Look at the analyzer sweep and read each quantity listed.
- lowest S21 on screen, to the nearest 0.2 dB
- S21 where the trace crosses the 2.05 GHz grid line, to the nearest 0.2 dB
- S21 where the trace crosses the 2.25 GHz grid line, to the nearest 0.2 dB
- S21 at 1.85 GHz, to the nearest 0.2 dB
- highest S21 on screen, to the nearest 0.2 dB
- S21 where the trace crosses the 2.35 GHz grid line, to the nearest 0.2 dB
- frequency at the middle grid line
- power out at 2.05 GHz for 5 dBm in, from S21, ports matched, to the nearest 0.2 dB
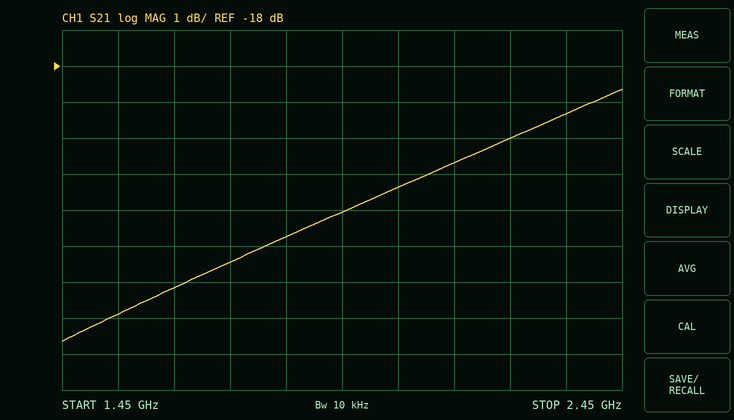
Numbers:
-25.6 dB
-21.4 dB
-20.0 dB
-22.8 dB
-18.6 dB
-19.4 dB
1.95 GHz
-16.4 dBm
